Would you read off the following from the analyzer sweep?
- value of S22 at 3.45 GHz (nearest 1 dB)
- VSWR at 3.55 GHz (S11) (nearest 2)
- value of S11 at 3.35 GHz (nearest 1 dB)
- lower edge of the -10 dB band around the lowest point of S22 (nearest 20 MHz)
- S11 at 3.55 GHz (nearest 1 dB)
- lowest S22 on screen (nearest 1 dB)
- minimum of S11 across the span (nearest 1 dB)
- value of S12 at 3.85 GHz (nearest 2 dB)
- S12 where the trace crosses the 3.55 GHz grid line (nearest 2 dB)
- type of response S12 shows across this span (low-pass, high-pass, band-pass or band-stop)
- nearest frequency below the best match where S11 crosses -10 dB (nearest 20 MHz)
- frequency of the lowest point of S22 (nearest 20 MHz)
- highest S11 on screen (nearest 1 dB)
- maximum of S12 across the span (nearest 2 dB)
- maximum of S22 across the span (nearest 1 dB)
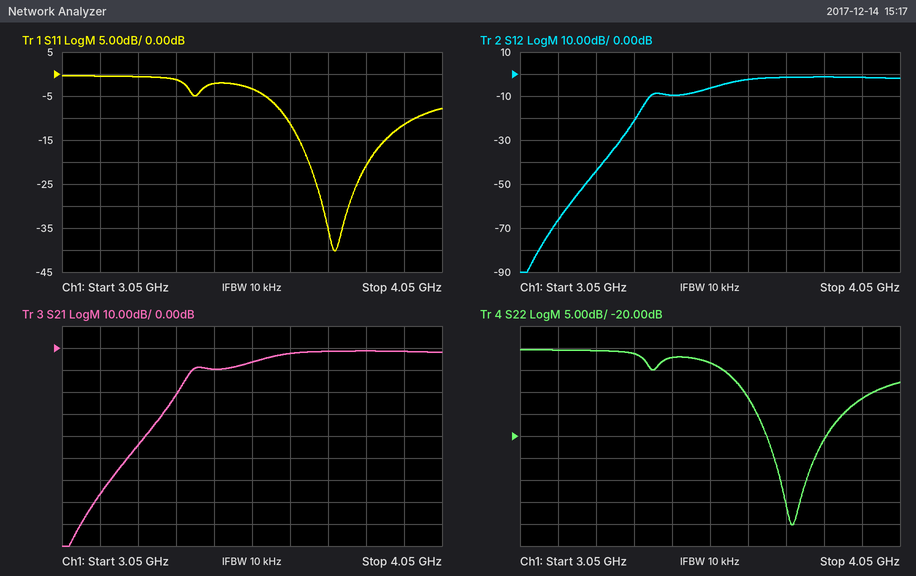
-2 dB
6
-1 dB
3.64 GHz
-3 dB
-40 dB
-40 dB
-2 dB
-6 dB
high-pass
3.64 GHz
3.76 GHz
0 dB
-2 dB
0 dB
